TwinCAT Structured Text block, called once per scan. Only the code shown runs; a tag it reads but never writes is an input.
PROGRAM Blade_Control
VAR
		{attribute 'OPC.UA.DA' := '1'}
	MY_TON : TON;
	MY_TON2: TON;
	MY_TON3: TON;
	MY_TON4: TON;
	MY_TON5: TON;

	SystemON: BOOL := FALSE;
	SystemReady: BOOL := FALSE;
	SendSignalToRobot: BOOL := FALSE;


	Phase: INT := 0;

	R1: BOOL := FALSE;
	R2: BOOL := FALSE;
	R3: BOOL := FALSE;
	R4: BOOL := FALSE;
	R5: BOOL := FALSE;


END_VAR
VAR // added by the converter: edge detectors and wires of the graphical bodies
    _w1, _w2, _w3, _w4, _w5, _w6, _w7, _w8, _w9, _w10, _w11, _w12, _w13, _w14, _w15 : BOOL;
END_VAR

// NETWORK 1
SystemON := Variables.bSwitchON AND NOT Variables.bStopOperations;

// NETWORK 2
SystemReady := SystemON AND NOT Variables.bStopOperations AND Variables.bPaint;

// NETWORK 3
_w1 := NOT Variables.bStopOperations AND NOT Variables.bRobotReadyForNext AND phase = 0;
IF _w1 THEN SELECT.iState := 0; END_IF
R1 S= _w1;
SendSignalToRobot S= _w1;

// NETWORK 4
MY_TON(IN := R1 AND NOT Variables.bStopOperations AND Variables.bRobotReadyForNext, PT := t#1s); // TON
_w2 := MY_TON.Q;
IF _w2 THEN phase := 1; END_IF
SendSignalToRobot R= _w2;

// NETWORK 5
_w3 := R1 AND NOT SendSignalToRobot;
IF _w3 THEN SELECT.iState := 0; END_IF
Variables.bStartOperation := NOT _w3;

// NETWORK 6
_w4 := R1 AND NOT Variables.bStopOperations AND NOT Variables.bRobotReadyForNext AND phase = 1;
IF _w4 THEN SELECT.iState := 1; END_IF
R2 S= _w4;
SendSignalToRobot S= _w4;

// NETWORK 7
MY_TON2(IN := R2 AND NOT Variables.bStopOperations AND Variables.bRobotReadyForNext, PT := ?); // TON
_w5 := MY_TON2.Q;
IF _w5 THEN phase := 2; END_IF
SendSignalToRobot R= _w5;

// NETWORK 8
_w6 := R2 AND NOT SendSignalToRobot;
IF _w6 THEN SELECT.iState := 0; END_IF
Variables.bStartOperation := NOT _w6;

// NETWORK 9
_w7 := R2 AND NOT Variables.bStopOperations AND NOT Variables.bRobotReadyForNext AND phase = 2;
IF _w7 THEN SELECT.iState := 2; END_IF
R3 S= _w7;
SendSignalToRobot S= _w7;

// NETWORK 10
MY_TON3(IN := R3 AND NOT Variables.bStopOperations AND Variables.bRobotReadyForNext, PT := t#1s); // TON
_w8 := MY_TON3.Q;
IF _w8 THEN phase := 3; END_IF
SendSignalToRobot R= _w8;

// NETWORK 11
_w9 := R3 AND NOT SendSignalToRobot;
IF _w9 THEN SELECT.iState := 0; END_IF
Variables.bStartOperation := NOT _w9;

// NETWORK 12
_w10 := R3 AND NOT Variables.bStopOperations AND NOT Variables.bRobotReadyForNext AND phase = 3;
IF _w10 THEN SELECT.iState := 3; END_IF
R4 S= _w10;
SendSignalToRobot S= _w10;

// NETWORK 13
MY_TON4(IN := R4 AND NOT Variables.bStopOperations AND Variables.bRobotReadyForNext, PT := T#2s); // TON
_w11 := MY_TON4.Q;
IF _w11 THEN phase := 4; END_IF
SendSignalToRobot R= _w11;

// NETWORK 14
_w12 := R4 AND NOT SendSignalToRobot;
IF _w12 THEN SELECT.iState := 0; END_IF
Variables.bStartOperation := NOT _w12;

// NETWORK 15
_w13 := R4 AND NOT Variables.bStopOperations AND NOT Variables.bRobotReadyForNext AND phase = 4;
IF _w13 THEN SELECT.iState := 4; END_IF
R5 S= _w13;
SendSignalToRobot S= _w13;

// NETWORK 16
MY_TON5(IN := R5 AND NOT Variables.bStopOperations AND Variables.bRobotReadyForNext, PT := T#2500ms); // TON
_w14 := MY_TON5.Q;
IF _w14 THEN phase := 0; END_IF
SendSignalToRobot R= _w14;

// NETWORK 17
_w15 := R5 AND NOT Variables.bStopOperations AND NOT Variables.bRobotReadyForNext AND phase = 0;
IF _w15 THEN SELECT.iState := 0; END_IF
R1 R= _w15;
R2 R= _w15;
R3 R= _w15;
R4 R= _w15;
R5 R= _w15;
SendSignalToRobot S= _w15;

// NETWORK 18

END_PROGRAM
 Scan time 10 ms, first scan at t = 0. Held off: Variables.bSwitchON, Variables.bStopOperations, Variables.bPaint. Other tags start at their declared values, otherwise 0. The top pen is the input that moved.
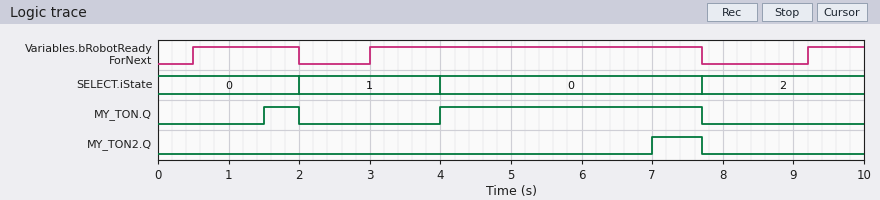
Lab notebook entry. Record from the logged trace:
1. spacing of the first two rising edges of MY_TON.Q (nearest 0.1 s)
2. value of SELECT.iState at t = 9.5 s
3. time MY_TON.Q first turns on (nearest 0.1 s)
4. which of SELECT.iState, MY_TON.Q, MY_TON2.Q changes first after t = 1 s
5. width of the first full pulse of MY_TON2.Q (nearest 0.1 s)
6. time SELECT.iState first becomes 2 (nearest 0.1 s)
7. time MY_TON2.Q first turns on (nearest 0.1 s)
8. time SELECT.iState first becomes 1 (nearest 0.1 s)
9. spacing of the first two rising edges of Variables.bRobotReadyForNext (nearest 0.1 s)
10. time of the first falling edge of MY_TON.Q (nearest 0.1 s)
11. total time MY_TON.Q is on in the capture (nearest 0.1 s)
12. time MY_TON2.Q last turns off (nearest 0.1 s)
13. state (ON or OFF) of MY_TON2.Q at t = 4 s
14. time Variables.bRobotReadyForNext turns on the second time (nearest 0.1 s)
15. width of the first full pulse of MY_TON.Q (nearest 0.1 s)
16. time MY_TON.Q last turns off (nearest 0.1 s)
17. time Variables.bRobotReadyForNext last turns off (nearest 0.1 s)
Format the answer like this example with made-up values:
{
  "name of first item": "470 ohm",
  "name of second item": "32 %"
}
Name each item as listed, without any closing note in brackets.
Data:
{
  "spacing of the first two rising edges of MY_TON.Q": "2.5 s",
  "value of SELECT.iState at t = 9.5 s": "2",
  "time MY_TON.Q first turns on": "1.5 s",
  "which of SELECT.iState, MY_TON.Q, MY_TON2.Q changes first after t = 1 s": "MY_TON.Q",
  "width of the first full pulse of MY_TON2.Q": "0.7 s",
  "time SELECT.iState first becomes 2": "7.7 s",
  "time MY_TON2.Q first turns on": "7.0 s",
  "time SELECT.iState first becomes 1": "2.0 s",
  "spacing of the first two rising edges of Variables.bRobotReadyForNext": "2.5 s",
  "time of the first falling edge of MY_TON.Q": "2.0 s",
  "total time MY_TON.Q is on in the capture": "4.2 s",
  "time MY_TON2.Q last turns off": "7.7 s",
  "state (ON or OFF) of MY_TON2.Q at t = 4 s": "OFF",
  "time Variables.bRobotReadyForNext turns on the second time": "3.0 s",
  "width of the first full pulse of MY_TON.Q": "0.5 s",
  "time MY_TON.Q last turns off": "7.7 s",
  "time Variables.bRobotReadyForNext last turns off": "7.7 s"
}
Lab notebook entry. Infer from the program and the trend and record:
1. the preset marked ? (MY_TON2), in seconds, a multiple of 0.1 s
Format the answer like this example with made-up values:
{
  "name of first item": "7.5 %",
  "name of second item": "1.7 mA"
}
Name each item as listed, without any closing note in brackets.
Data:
{
  "the preset marked ? (MY_TON2), in seconds, a multiple of 0.1 s": "4.0 s"
}
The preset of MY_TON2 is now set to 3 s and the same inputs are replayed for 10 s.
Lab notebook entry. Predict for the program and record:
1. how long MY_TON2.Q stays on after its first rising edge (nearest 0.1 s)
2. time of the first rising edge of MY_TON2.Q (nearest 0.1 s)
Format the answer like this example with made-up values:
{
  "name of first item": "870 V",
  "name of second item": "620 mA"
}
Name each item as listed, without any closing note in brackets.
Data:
{
  "how long MY_TON2.Q stays on after its first rising edge": "1.7 s",
  "time of the first rising edge of MY_TON2.Q": "6.0 s"
}
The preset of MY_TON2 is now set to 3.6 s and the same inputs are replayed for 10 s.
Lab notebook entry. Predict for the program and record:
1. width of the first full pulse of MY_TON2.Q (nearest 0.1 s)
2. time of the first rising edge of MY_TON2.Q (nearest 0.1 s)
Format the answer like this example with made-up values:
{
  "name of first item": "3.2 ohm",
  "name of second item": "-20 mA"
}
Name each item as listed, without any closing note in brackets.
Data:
{
  "width of the first full pulse of MY_TON2.Q": "1.1 s",
  "time of the first rising edge of MY_TON2.Q": "6.6 s"
}
